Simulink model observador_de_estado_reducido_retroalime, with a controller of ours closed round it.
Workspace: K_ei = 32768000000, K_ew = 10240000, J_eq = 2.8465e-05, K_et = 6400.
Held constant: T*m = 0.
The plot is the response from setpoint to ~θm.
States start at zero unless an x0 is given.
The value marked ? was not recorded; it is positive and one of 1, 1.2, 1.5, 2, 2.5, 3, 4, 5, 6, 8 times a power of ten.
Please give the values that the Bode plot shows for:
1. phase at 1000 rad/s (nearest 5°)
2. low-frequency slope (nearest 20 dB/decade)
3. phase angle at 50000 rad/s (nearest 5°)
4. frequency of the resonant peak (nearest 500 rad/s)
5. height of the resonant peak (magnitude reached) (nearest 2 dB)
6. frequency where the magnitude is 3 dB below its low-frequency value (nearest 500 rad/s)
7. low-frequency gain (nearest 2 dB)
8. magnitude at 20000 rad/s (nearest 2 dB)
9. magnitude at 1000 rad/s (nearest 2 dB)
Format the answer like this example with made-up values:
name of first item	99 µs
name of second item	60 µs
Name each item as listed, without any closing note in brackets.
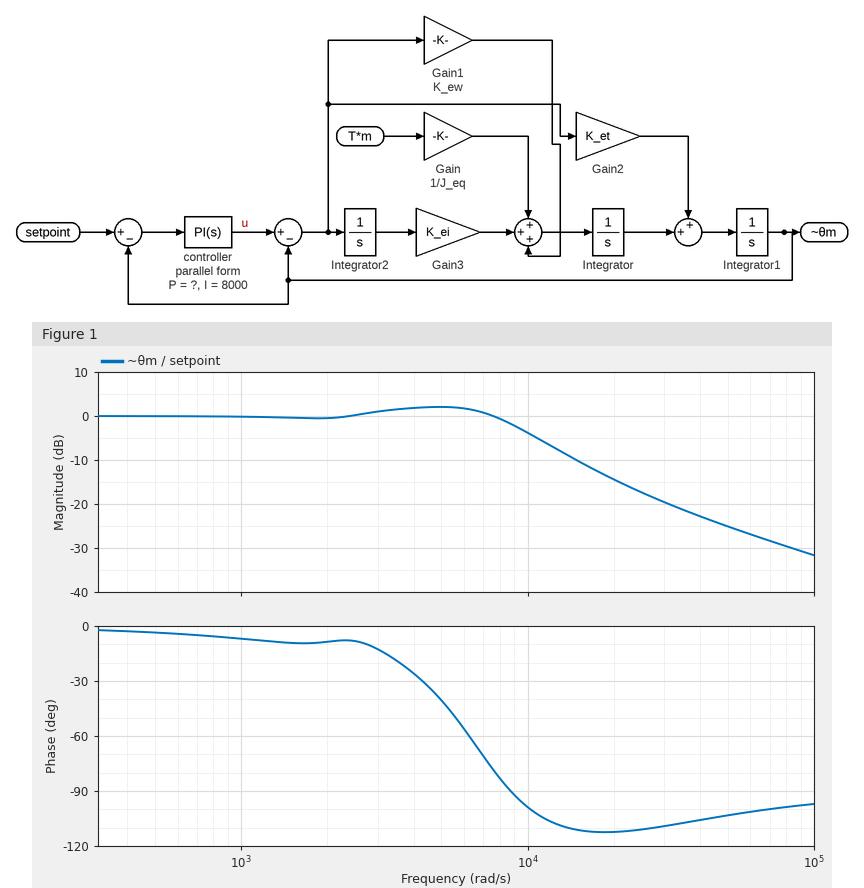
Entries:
phase at 1000 rad/s	-5°
low-frequency slope	0 dB/decade
phase angle at 50000 rad/s	-105°
frequency of the resonant peak	5000 rad/s
height of the resonant peak (magnitude reached)	2 dB
frequency where the magnitude is 3 dB below its low-frequency value	9500 rad/s
low-frequency gain	0 dB
magnitude at 20000 rad/s	-14 dB
magnitude at 1000 rad/s	0 dB
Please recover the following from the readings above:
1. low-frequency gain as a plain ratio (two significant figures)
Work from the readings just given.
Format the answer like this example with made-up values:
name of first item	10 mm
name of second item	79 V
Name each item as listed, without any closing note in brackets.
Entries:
low-frequency gain as a plain ratio	1.0
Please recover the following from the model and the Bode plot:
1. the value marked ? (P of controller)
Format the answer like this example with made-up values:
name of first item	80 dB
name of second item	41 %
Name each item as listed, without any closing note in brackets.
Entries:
the value marked ?	0.4
